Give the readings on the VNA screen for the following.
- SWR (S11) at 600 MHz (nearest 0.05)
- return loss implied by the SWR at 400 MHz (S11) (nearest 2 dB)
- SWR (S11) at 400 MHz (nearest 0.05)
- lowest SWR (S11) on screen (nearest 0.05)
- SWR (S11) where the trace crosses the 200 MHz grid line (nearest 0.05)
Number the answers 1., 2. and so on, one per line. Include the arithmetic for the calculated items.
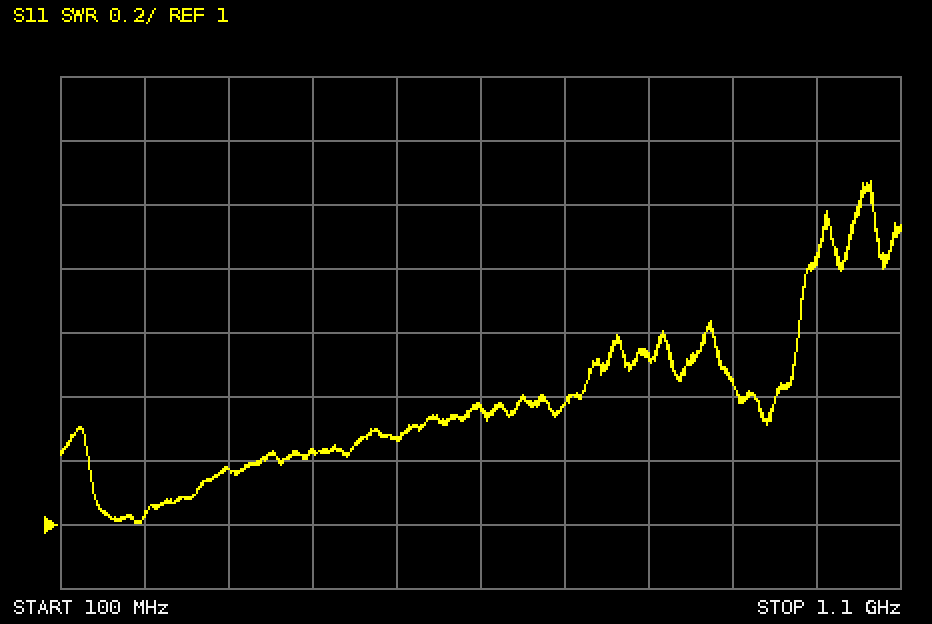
1. 1.35
2. −20 log10((1.25 − 1)/(1.25 + 1)) ≈ 19.1 dB, so 20 dB to the nearest 2 dB
3. 1.25
4. 1.00
5. 1.05
